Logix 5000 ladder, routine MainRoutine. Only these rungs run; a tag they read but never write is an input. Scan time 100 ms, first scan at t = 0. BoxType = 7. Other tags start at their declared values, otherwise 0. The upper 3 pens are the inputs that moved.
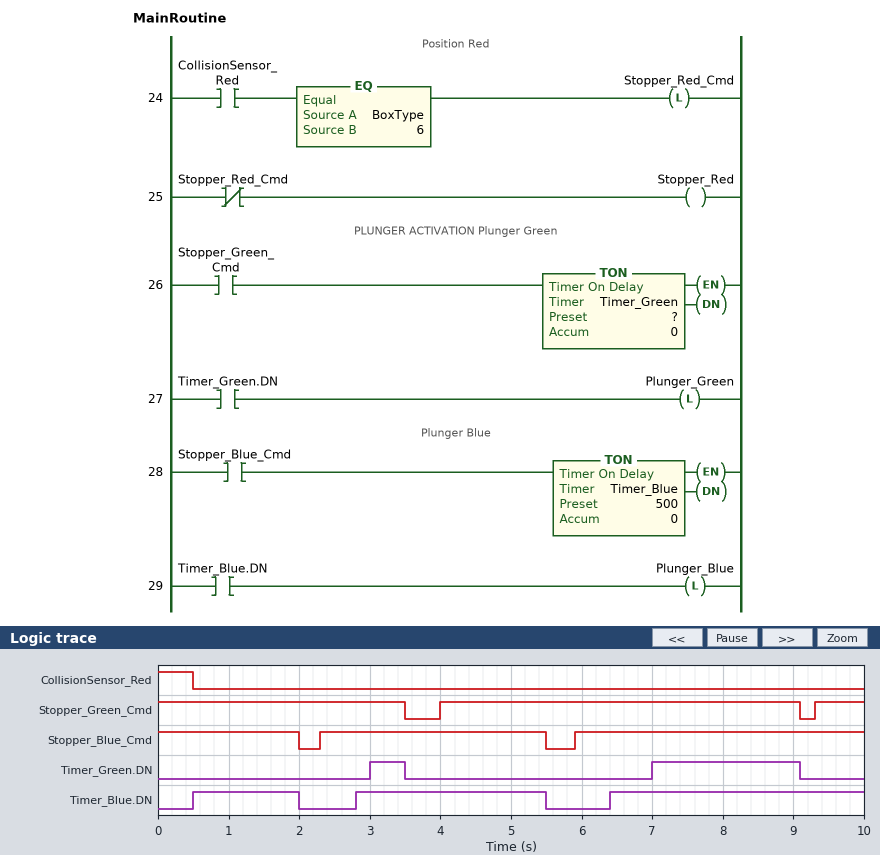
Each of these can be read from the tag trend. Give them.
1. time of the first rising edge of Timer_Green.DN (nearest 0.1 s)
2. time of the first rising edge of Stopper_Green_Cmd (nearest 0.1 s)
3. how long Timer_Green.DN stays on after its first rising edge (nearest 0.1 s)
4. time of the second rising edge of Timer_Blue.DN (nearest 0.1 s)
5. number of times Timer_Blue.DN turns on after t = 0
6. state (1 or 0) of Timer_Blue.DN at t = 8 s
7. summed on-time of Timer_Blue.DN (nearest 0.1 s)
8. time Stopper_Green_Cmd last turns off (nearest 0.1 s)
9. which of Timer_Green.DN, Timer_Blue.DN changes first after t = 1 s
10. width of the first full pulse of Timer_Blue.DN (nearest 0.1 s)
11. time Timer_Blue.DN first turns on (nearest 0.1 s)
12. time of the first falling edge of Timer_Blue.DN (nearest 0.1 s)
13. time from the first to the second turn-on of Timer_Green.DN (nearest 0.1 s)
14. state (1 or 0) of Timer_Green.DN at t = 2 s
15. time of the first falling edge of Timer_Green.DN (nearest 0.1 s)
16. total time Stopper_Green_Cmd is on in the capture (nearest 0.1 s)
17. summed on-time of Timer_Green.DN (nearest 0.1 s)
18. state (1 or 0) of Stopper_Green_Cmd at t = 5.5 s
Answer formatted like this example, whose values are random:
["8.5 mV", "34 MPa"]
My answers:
["3.0 s", "4.0 s", "0.5 s", "2.8 s", "3", "1", "7.8 s", "9.1 s", "Timer_Blue.DN", "1.5 s", "0.5 s", "2.0 s", "4.0 s", "0", "3.5 s", "9.3 s", "2.6 s", "1"]
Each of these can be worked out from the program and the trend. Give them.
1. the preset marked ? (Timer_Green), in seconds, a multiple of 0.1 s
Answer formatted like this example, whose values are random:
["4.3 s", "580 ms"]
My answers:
["3.0 s"]
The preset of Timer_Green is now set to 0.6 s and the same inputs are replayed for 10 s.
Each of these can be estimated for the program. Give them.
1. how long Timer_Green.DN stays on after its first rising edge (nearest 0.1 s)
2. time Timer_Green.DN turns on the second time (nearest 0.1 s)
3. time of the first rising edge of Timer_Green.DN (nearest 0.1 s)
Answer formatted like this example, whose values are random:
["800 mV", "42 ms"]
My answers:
["2.9 s", "4.6 s", "0.6 s"]
